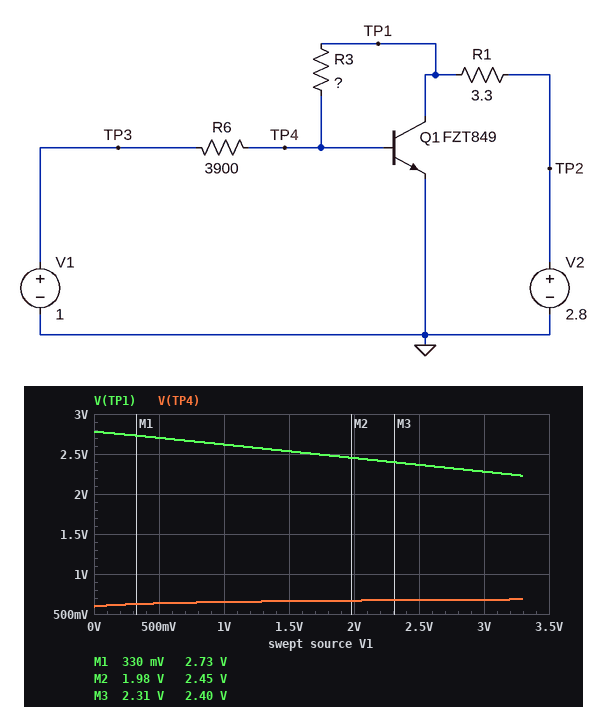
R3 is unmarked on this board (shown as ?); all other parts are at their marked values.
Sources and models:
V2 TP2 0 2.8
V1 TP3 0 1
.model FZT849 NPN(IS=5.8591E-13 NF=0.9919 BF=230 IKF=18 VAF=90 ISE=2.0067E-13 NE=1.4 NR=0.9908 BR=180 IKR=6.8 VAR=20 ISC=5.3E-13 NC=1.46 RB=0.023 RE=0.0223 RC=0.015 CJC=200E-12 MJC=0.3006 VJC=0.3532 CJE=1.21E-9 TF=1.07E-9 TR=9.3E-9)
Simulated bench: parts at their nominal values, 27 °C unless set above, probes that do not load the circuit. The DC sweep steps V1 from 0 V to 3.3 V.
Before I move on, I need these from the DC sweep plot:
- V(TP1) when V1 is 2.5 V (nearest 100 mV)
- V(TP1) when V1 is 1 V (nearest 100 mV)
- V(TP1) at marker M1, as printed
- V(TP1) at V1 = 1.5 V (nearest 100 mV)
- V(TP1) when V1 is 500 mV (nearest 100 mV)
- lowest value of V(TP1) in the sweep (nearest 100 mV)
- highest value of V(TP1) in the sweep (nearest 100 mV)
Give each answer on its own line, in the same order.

2.4 V
2.6 V
2.73 V
2.5 V
2.7 V
2.2 V
2.8 V
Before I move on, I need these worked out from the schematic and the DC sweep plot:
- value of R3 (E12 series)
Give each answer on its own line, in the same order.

12 kΩ
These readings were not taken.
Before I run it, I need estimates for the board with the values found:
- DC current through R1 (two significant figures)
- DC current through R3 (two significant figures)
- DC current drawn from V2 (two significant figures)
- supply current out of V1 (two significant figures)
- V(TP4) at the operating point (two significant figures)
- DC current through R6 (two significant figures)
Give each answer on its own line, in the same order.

55 mA
160 µA
55 mA
90 µA
650 mV
90 µA
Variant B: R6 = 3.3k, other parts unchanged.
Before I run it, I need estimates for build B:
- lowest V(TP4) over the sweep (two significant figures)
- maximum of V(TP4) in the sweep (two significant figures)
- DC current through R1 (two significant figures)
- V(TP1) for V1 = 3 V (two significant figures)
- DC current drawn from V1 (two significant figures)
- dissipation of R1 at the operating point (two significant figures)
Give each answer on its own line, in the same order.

570 mV
690 mV
58 mA
2.2 V
110 µA
11 mW
